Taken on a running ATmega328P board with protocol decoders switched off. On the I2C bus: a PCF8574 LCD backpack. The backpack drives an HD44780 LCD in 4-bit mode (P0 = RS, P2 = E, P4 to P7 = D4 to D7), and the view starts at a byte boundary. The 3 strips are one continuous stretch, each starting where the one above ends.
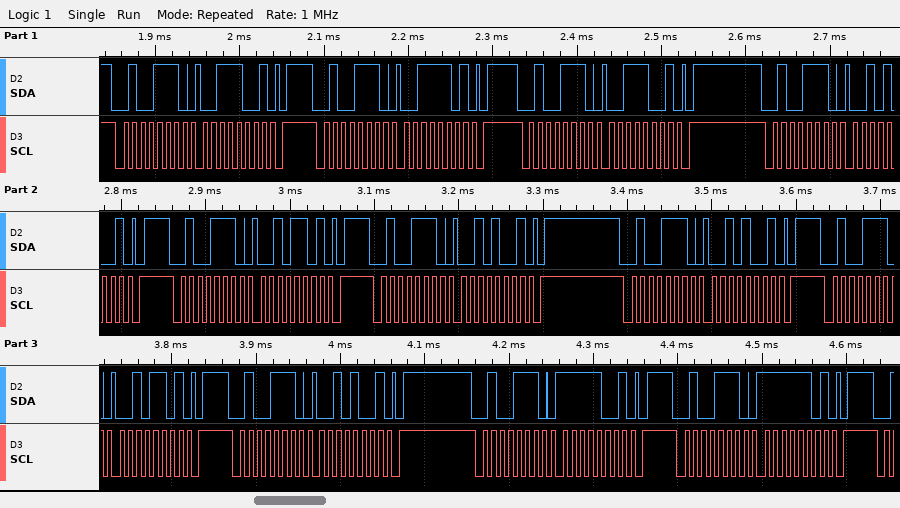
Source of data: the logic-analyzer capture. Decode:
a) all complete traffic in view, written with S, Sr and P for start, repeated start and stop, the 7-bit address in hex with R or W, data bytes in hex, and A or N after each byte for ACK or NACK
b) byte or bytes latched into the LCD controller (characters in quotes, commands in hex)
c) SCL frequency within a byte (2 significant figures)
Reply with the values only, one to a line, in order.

S 27W A 39 A P S 27W A 3D A P S 27W A 39 A P S 27W A 29 A P S 27W A 2D A P S 27W A 29 A P S 27W A 29 A P S 27W A 2D A P S 27W A 29 A P S 27W A F9 A P S 27W A FD A P
'2'
100 kHz
